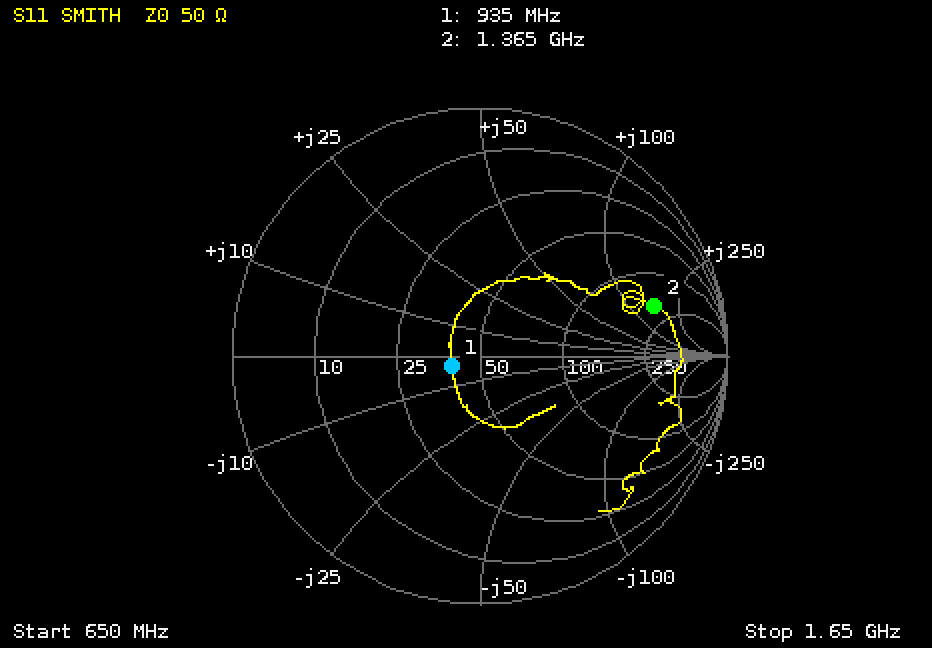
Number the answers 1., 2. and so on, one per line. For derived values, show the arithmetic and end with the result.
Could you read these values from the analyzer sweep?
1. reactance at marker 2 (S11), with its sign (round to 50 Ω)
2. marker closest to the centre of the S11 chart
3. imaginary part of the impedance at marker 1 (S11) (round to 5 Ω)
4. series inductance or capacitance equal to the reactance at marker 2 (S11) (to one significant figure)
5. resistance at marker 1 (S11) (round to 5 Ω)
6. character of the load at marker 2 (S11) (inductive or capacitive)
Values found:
1. +150 Ω
2. marker 1
3. -5 Ω
4. L = 150 Ω/(2π × 1.365 GHz) ≈ 17.5 nH, so 20 nH to one significant figure
5. 40 Ω
6. inductive
